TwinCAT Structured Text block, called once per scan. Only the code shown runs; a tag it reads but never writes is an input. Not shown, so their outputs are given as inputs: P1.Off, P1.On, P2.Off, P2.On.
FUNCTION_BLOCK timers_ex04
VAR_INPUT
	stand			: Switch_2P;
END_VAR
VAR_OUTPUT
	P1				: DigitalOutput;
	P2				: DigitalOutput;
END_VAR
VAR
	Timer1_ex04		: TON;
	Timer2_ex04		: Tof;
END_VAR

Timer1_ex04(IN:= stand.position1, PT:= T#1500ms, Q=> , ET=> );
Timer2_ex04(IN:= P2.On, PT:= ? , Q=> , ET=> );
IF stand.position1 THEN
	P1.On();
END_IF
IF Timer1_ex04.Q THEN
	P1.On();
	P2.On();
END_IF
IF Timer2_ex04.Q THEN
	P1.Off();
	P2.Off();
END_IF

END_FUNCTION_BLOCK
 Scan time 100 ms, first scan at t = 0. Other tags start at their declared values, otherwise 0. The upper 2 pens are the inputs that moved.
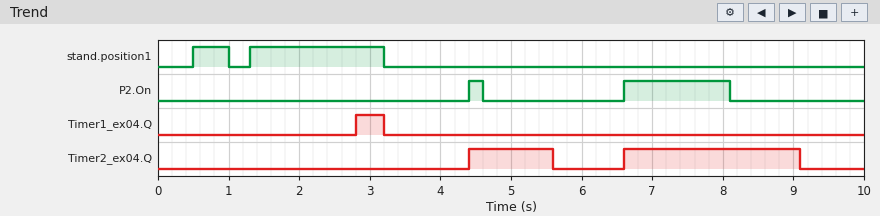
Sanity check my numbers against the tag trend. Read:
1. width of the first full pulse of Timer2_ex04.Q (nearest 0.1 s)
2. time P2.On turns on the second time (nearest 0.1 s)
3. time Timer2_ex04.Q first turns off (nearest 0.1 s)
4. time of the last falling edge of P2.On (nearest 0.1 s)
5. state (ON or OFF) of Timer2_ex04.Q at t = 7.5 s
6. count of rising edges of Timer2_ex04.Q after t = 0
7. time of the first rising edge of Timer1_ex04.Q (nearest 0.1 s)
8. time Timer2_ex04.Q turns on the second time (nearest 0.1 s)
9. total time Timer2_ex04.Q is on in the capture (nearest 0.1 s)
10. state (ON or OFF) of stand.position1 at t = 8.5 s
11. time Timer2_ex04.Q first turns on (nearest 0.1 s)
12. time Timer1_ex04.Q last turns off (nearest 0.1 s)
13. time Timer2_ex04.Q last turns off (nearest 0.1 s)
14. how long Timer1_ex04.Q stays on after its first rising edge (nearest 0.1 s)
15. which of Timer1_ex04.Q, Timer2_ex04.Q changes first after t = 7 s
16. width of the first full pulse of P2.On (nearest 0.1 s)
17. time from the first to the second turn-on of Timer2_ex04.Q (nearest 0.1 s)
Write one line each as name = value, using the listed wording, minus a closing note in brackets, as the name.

width of the first full pulse of Timer2_ex04.Q = 1.2 s
time P2.On turns on the second time = 6.6 s
time Timer2_ex04.Q first turns off = 5.6 s
time of the last falling edge of P2.On = 8.1 s
state (ON or OFF) of Timer2_ex04.Q at t = 7.5 s = ON
count of rising edges of Timer2_ex04.Q after t = 0 = 2
time of the first rising edge of Timer1_ex04.Q = 2.8 s
time Timer2_ex04.Q turns on the second time = 6.6 s
total time Timer2_ex04.Q is on in the capture = 3.7 s
state (ON or OFF) of stand.position1 at t = 8.5 s = OFF
time Timer2_ex04.Q first turns on = 4.4 s
time Timer1_ex04.Q last turns off = 3.2 s
time Timer2_ex04.Q last turns off = 9.1 s
how long Timer1_ex04.Q stays on after its first rising edge = 0.4 s
which of Timer1_ex04.Q, Timer2_ex04.Q changes first after t = 7 s = Timer2_ex04.Q
width of the first full pulse of P2.On = 0.2 s
time from the first to the second turn-on of Timer2_ex04.Q = 2.2 s
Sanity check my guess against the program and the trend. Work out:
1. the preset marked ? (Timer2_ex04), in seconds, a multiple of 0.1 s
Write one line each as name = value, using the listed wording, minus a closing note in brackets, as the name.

the preset marked ? (Timer2_ex04), in seconds, a multiple of 0.1 s = 1.0 s
